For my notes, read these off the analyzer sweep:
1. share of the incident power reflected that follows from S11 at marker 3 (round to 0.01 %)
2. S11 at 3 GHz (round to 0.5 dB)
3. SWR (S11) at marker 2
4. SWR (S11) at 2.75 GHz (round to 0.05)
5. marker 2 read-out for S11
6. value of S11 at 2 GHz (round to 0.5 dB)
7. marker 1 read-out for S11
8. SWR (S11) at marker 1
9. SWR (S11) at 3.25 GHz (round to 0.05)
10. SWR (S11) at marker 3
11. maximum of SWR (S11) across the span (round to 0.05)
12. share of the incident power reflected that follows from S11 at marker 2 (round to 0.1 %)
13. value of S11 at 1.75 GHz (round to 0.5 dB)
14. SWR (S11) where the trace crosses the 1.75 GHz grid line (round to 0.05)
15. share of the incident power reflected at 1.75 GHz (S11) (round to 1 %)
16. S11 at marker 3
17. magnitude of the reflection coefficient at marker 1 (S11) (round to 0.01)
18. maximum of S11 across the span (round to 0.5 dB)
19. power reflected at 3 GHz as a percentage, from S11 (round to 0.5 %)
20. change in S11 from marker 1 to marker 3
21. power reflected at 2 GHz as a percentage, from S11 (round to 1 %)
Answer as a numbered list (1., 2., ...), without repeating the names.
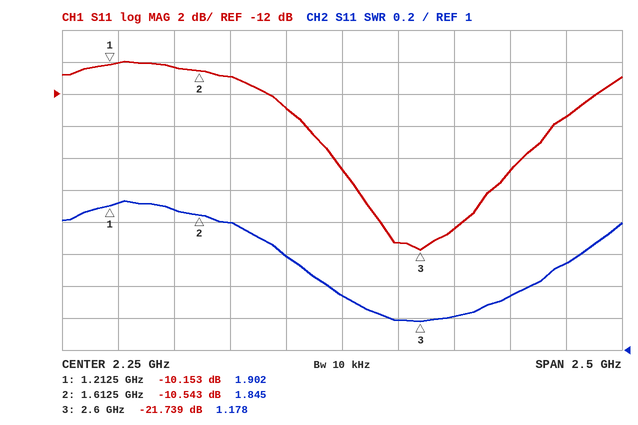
1. 0.67 %
2. -17.0 dB
3. 1.845
4. 1.20
5. -10.543 dB
6. -13.0 dB
7. -10.153 dB
8. 1.902
9. 1.55
10. 1.178
11. 1.95
12. 8.8 %
13. -11.0 dB
14. 1.80
15. 8 %
16. -21.739 dB
17. 0.31
18. -10.0 dB
19. 2.0 %
20. -11.586 dB
21. 5 %
